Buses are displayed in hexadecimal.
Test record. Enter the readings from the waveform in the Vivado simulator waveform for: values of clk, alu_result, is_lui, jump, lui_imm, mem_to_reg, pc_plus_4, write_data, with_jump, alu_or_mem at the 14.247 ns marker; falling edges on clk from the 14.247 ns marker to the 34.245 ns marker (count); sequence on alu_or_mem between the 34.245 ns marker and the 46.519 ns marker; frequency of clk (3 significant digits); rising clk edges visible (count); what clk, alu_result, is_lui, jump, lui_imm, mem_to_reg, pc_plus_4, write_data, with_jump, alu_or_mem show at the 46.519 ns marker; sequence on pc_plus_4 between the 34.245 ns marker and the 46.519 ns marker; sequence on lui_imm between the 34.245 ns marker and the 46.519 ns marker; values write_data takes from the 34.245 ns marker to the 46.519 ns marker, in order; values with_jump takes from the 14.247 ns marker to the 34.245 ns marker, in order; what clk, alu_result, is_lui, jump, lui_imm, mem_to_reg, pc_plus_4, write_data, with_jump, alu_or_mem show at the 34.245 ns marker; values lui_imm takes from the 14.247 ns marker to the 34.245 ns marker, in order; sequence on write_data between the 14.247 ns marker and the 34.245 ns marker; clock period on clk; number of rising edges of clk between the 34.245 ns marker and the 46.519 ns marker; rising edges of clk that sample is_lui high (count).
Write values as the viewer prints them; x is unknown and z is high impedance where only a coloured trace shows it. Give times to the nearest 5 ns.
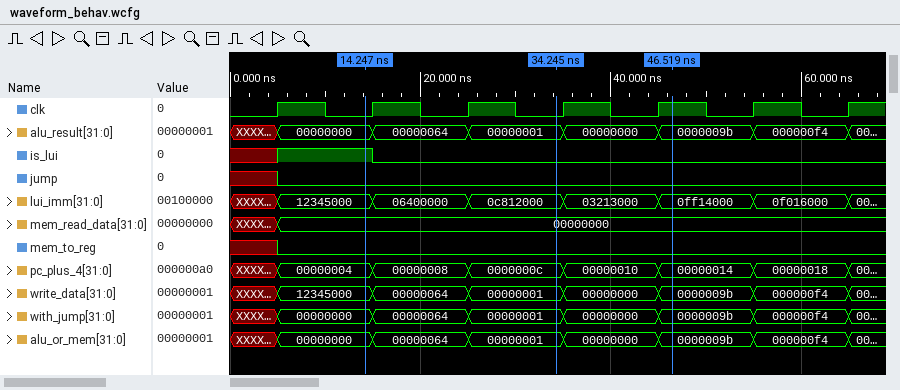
clk=0, alu_result=00000000, is_lui=1, jump=0, lui_imm=12345000, mem_to_reg=0, pc_plus_4=00000004, write_data=12345000, with_jump=00000000, alu_or_mem=00000000
2
00000001, 00000000, 0000009b
100 MHz
7
clk=1, alu_result=0000009b, is_lui=0, jump=0, lui_imm=0ff14000, mem_to_reg=0, pc_plus_4=00000014, write_data=0000009b, with_jump=0000009b, alu_or_mem=0000009b
0000000c, 00000010, 00000014
0c812000, 03213000, 0ff14000
00000001, 00000000, 0000009b
00000000, 00000064, 00000001
clk=0, alu_result=00000001, is_lui=0, jump=0, lui_imm=0c812000, mem_to_reg=0, pc_plus_4=0000000c, write_data=00000001, with_jump=00000001, alu_or_mem=00000001
12345000, 06400000, 0c812000
12345000, 00000064, 00000001
10 ns
2
1
